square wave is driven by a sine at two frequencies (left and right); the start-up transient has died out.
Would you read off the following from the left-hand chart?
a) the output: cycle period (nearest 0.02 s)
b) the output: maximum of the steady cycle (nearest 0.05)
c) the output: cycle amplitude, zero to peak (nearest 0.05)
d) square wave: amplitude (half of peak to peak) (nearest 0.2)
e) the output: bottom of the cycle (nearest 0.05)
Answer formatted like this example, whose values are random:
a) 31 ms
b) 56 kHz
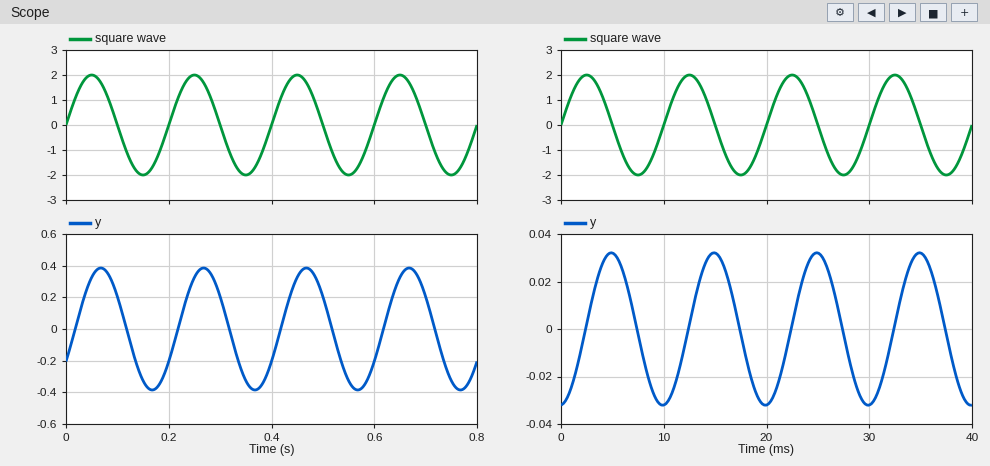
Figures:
a) 0.20 s
b) 0.40
c) 0.40
d) 2.0
e) -0.40
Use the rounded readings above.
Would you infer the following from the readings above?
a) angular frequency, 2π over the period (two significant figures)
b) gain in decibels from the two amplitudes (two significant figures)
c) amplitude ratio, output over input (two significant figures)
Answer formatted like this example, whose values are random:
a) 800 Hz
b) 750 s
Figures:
a) 31 rad/s
b) -14 dB
c) 0.20
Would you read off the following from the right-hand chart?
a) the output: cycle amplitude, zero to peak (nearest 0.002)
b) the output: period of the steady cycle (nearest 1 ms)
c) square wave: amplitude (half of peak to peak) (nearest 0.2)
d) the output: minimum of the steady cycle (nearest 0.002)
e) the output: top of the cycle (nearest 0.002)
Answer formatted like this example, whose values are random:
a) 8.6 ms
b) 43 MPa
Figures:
a) 0.032
b) 10 ms
c) 2.0
d) -0.032
e) 0.032
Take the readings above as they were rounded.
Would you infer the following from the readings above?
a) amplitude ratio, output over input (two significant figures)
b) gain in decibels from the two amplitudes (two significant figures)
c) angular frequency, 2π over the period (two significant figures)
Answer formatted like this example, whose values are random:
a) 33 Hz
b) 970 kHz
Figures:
a) 0.016
b) -36 dB
c) 0.63 rad/ms
